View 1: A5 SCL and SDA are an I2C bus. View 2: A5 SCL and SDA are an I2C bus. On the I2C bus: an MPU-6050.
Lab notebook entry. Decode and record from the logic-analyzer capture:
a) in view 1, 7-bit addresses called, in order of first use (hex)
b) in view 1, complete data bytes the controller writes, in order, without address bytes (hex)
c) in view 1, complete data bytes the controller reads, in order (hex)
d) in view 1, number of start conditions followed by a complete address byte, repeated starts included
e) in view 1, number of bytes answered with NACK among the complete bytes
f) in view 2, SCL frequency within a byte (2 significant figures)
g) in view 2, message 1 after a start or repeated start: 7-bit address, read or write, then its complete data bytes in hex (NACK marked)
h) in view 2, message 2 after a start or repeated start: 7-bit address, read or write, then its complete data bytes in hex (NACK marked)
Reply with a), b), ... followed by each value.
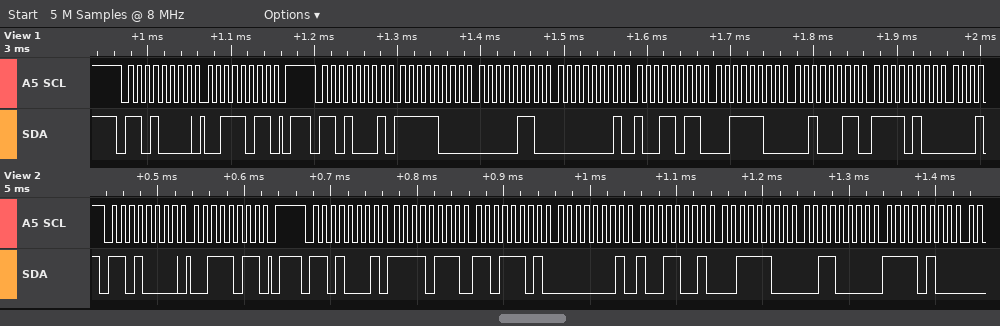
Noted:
a) 0x68
b) 3B
c) F8 06 01 9B 3C 23 F4
d) 2
e) 0
f) 100 kHz
g) 0x68 write: 3B
h) 0x68 read: F7 DD 01 99 3C 30 F4
